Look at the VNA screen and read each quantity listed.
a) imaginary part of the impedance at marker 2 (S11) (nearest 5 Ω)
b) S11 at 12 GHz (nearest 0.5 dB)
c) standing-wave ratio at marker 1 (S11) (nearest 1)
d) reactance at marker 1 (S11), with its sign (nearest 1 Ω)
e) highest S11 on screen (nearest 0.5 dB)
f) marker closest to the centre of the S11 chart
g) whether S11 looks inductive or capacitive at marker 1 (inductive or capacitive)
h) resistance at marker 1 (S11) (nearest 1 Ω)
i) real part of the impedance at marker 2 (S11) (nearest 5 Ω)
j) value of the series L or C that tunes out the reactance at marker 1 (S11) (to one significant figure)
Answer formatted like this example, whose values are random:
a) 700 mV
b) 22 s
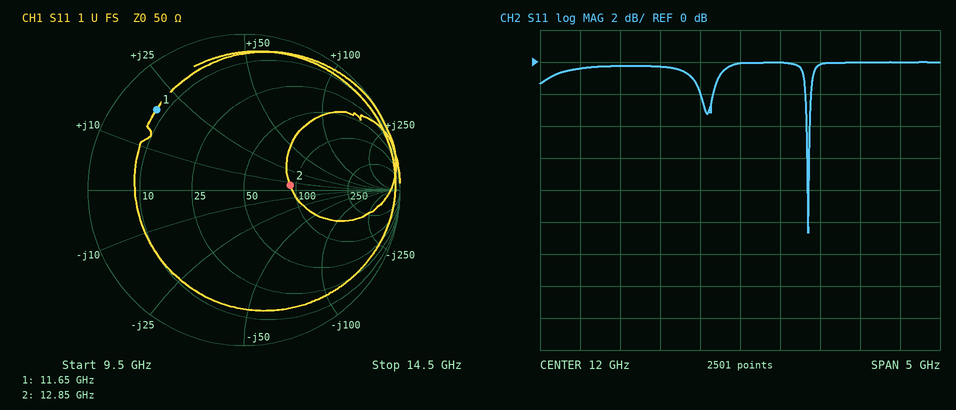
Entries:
a) +5 Ω
b) 0.0 dB
c) 7
d) +19 Ω
e) 0.0 dB
f) marker 2
g) inductive
h) 8 Ω
i) 90 Ω
j) 700 fF
